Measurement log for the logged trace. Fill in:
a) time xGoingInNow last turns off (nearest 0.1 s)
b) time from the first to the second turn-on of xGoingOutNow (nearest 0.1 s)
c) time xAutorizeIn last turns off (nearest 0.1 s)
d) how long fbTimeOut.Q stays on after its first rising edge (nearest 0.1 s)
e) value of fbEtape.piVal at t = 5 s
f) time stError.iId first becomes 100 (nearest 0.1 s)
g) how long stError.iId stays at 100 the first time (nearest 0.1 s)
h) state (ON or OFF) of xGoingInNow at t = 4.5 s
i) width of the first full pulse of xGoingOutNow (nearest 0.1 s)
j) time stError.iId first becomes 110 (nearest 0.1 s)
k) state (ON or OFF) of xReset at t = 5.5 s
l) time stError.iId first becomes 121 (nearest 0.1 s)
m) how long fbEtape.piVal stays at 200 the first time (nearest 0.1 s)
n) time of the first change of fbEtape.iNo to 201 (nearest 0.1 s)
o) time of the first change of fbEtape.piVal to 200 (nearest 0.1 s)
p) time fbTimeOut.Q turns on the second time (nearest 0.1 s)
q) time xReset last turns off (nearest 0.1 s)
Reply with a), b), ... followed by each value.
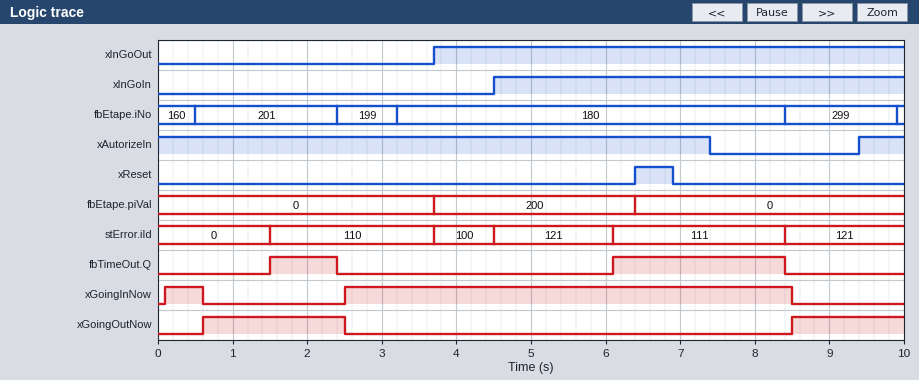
a) 8.5 s
b) 7.9 s
c) 7.4 s
d) 0.9 s
e) 200
f) 3.7 s
g) 0.8 s
h) ON
i) 1.9 s
j) 1.5 s
k) OFF
l) 4.5 s
m) 2.7 s
n) 0.5 s
o) 3.7 s
p) 6.1 s
q) 6.9 s
